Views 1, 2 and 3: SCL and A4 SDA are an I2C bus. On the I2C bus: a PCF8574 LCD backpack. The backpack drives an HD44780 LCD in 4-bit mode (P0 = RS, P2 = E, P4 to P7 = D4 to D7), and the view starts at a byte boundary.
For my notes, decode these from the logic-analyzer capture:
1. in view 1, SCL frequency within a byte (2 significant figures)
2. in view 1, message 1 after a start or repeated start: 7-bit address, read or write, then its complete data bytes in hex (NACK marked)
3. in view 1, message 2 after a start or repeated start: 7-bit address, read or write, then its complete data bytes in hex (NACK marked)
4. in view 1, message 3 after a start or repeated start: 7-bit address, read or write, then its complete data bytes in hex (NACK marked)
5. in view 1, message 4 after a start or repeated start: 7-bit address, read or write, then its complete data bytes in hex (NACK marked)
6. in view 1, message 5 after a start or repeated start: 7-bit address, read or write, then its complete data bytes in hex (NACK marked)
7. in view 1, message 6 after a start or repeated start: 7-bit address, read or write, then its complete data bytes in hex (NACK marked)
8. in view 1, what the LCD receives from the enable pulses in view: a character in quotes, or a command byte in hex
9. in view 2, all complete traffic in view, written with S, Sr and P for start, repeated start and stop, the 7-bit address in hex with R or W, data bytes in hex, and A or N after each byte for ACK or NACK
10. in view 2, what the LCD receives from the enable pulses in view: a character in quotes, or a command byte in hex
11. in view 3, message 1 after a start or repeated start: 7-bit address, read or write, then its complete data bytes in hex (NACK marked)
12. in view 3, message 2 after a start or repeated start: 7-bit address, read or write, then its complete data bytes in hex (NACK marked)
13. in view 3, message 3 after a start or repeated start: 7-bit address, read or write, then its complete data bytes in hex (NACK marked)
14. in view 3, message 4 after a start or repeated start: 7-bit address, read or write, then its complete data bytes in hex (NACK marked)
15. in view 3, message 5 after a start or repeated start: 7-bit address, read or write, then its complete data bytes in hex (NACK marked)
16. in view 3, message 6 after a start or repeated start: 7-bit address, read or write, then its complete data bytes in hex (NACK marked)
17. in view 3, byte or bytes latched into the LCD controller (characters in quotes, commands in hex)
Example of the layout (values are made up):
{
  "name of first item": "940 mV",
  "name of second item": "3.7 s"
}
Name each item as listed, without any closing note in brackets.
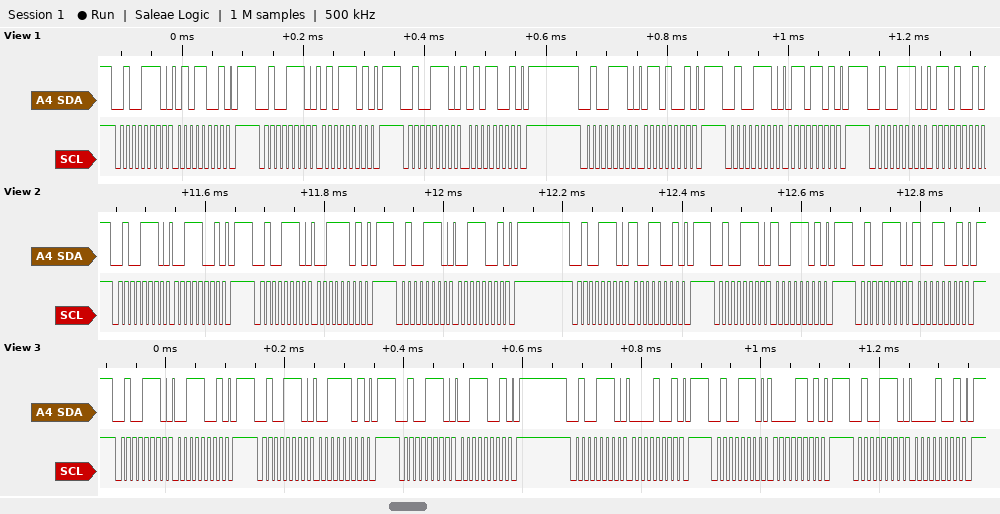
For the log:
{
  "in view 1, SCL frequency within a byte": "100 kHz",
  "in view 1, message 1 after a start or repeated start: 7-bit address, read or write, then its complete data bytes in hex": "0x27 write: 59",
  "in view 1, message 2 after a start or repeated start: 7-bit address, read or write, then its complete data bytes in hex": "0x27 write: 5D",
  "in view 1, message 3 after a start or repeated start: 7-bit address, read or write, then its complete data bytes in hex": "0x27 write: 59",
  "in view 1, message 4 after a start or repeated start: 7-bit address, read or write, then its complete data bytes in hex": "0x27 write: 69",
  "in view 1, message 5 after a start or repeated start: 7-bit address, read or write, then its complete data bytes in hex": "0x27 write: 6D",
  "in view 1, message 6 after a start or repeated start: 7-bit address, read or write, then its complete data bytes in hex": "0x27 write: 69",
  "in view 1, what the LCD receives from the enable pulses in view: a character in quotes, or a command byte in hex": "'V'",
  "in view 2, all complete traffic in view, written with S, Sr and P for start, repeated start and stop, the 7-bit address in hex with R or W, data bytes in hex, and A or N after each byte for ACK or NACK": "S 27W A 39 A P S 27W A 3D A P S 27W A 39 A P S 27W A 99 A P S 27W A 9D A P S 27W A 99 A P",
  "in view 2, what the LCD receives from the enable pulses in view: a character in quotes, or a command byte in hex": "'9'",
  "in view 3, message 1 after a start or repeated start: 7-bit address, read or write, then its complete data bytes in hex": "0x27 write: 39",
  "in view 3, message 2 after a start or repeated start: 7-bit address, read or write, then its complete data bytes in hex": "0x27 write: 3D",
  "in view 3, message 3 after a start or repeated start: 7-bit address, read or write, then its complete data bytes in hex": "0x27 write: 39",
  "in view 3, message 4 after a start or repeated start: 7-bit address, read or write, then its complete data bytes in hex": "0x27 write: 09",
  "in view 3, message 5 after a start or repeated start: 7-bit address, read or write, then its complete data bytes in hex": "0x27 write: 0D",
  "in view 3, message 6 after a start or repeated start: 7-bit address, read or write, then its complete data bytes in hex": "0x27 write: 09",
  "in view 3, byte or bytes latched into the LCD controller": "'0'"
}
